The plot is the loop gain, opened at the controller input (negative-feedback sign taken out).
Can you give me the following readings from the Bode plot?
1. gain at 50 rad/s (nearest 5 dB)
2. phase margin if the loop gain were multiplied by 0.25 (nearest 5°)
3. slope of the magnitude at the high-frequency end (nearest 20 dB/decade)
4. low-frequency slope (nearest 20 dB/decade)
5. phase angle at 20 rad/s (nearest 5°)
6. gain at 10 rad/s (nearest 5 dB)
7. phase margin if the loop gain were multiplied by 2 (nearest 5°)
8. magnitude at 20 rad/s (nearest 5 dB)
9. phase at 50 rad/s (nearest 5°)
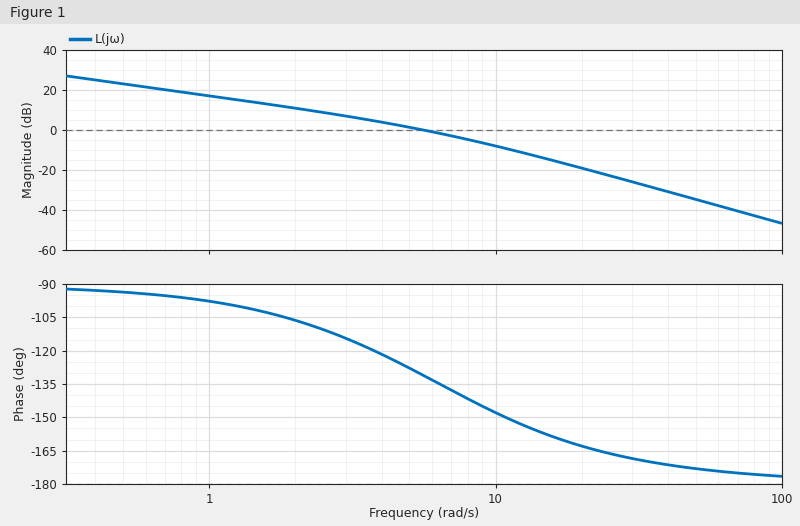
-35 dB
75°
-40 dB/decade
-20 dB/decade
-165°
-10 dB
35°
-20 dB
-175°
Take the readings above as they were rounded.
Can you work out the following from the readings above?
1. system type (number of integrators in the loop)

1
